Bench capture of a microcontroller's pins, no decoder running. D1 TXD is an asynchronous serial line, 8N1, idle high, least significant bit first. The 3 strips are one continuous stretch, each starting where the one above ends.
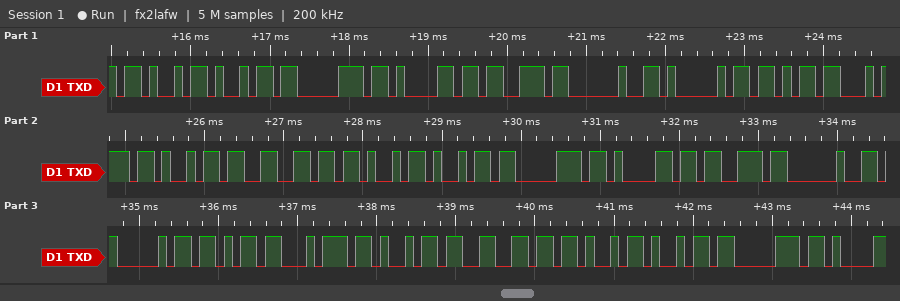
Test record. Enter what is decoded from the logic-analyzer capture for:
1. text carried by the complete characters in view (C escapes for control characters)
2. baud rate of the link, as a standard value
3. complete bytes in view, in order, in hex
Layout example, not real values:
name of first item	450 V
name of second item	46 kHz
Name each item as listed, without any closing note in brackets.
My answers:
text carried by the complete characters in view	"Kipas AktifKipas AktifKip"
baud rate of the link, as a standard value	9600 baud
complete bytes in view, in order, in hex	4B 69 70 61 73 20 41 6B 74 69 66 4B 69 70 61 73 20 41 6B 74 69 66 4B 69 70
